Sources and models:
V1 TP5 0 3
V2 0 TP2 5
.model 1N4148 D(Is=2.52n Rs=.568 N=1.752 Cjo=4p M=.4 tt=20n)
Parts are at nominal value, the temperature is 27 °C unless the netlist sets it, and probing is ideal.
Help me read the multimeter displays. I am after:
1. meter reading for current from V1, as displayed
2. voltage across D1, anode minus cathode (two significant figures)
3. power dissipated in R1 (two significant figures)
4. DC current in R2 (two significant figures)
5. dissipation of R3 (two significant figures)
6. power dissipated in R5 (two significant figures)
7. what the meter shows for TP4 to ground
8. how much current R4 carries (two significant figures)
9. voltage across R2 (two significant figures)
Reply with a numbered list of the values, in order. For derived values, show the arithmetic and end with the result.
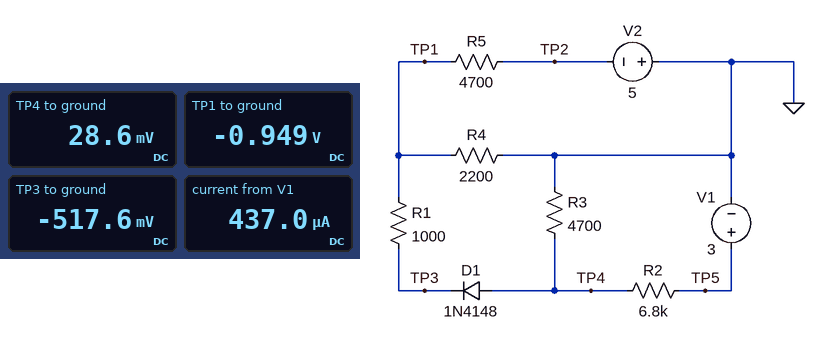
1. 437.0 µA
2. 28.6 mV - (-517.6 mV) = 550 mV
3. (-517.6 mV - (-949 mV))^2 / 1 kΩ = 190 µW
4. (3 V - 28.6 mV) / 6.8 kΩ = 440 µA
5. (28.6 mV)^2 / 4.7 kΩ = 170 nW
6. (-949 mV - (-5 V))^2 / 4.7 kΩ = 3.5 mW
7. 28.6 mV
8. (0 V - (-949 mV)) / 2.2 kΩ = 430 µA
9. 3 V - 28.6 mV = 3.0 V
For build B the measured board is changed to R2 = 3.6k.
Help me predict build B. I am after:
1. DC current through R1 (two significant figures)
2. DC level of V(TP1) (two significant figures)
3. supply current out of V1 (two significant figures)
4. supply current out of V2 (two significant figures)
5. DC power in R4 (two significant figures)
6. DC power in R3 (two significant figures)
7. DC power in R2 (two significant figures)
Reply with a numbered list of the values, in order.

1. 600 µA
2. -690 mV
3. 700 µA
4. 920 µA
5. 220 µW
6. 47 µW
7. 1.8 mW
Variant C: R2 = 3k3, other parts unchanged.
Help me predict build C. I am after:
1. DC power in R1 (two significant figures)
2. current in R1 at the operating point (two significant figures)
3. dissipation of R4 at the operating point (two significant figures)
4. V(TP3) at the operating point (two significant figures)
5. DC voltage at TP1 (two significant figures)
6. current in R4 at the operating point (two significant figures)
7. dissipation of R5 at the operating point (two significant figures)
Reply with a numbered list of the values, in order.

1. 400 µW
2. 630 µA
3. 190 µW
4. -21 mV
5. -650 mV
6. 300 µA
7. 4.0 mW
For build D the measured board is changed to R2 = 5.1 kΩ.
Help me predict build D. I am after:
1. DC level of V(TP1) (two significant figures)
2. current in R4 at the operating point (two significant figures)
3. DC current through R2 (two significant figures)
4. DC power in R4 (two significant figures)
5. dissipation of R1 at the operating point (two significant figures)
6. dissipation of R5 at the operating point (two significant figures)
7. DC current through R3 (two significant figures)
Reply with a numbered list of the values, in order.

1. -840 mV
2. 380 µA
3. 550 µA
4. 320 µW
5. 250 µW
6. 3.7 mW
7. 45 µA
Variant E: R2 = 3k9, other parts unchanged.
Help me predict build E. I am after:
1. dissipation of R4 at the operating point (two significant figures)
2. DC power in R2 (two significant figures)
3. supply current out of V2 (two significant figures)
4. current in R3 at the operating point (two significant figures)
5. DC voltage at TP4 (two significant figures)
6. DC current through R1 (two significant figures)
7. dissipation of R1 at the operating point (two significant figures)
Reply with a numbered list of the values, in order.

1. 240 µW
2. 1.7 mW
3. 910 µA
4. 87 µA
5. 410 mV
6. 580 µA
7. 330 µW
